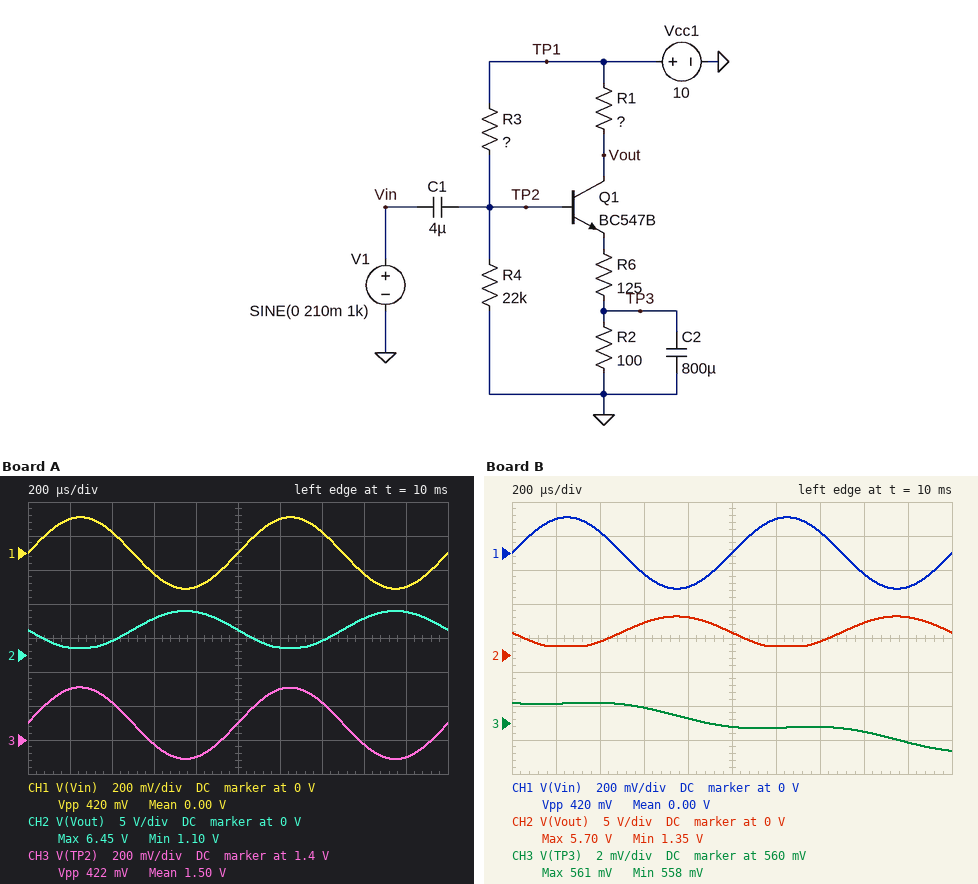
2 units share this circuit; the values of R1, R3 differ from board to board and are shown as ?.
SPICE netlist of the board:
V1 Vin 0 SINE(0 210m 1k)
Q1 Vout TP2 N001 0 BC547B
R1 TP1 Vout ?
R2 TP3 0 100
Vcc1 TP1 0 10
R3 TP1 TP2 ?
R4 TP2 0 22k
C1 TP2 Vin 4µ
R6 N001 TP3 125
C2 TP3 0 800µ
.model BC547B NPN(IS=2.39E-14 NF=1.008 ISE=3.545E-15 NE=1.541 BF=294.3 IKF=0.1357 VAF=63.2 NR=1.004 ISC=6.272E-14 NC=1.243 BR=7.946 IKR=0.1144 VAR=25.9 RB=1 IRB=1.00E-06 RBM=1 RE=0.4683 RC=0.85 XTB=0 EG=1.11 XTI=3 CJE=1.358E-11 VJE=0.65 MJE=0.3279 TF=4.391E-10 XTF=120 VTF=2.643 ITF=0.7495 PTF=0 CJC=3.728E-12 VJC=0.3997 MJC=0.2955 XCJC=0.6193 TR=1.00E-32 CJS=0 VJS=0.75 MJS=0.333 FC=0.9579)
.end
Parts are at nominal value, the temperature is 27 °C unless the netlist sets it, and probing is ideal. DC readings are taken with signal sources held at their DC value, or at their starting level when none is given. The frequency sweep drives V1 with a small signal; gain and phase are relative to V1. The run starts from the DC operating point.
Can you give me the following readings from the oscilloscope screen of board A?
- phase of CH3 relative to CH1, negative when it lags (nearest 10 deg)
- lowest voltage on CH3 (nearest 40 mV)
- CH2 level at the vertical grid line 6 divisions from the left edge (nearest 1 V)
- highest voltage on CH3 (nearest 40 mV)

0 deg
1.28 V
1 V
1.72 V
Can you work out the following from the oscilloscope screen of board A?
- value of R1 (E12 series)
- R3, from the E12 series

1.8 kΩ
100 kΩ
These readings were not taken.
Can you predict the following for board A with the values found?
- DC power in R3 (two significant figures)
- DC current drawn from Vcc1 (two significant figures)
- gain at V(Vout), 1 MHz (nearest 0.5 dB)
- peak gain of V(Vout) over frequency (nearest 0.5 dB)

710 µW
4.0 mA
22.5 dB
22.5 dB
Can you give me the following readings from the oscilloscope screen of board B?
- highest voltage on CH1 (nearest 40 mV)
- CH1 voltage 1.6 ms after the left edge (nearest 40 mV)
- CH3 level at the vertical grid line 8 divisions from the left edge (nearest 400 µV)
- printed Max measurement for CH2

200 mV
-120 mV
559.6 mV
5.70 V
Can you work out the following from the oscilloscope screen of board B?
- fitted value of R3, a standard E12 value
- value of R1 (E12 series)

68 kΩ
1.5 kΩ
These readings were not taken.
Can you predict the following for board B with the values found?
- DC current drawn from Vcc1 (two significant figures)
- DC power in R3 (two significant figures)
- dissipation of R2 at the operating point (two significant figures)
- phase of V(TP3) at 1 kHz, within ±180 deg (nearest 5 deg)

5.8 mA
950 µW
3.3 mW
-85 deg
